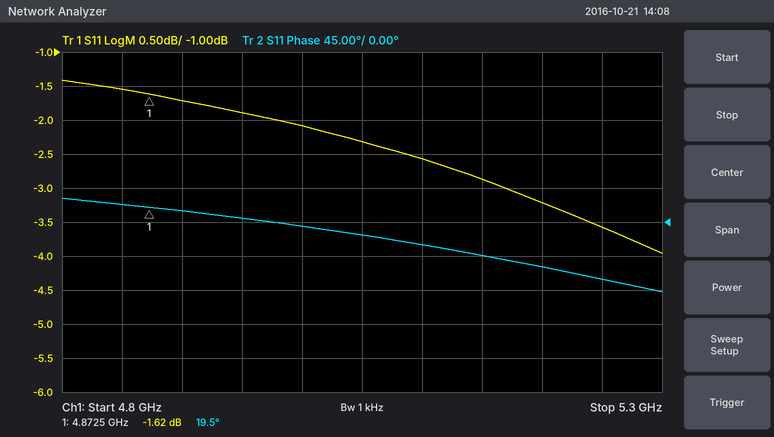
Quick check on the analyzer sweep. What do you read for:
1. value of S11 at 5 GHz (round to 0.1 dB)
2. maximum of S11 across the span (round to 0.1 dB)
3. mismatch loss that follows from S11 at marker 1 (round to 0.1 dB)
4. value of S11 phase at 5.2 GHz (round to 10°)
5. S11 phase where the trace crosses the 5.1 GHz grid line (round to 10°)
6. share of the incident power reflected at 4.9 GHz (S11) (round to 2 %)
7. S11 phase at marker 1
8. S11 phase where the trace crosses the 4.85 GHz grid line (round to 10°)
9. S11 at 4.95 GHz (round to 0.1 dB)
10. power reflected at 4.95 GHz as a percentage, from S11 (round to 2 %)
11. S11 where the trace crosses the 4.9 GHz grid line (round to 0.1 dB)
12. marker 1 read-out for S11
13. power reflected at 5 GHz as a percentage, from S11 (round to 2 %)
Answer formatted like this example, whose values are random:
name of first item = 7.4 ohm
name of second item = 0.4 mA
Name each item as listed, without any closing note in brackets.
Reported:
value of S11 at 5 GHz = -2.1 dB
maximum of S11 across the span = -1.4 dB
mismatch loss that follows from S11 at marker 1 = 5.1 dB
value of S11 phase at 5.2 GHz = -60°
S11 phase where the trace crosses the 5.1 GHz grid line = -30°
share of the incident power reflected at 4.9 GHz (S11) = 68 %
S11 phase at marker 1 = 19.5°
S11 phase where the trace crosses the 4.85 GHz grid line = 20°
S11 at 4.95 GHz = -1.9 dB
power reflected at 4.95 GHz as a percentage, from S11 = 64 %
S11 where the trace crosses the 4.9 GHz grid line = -1.7 dB
marker 1 read-out for S11 = -1.62 dB
power reflected at 5 GHz as a percentage, from S11 = 62 %
